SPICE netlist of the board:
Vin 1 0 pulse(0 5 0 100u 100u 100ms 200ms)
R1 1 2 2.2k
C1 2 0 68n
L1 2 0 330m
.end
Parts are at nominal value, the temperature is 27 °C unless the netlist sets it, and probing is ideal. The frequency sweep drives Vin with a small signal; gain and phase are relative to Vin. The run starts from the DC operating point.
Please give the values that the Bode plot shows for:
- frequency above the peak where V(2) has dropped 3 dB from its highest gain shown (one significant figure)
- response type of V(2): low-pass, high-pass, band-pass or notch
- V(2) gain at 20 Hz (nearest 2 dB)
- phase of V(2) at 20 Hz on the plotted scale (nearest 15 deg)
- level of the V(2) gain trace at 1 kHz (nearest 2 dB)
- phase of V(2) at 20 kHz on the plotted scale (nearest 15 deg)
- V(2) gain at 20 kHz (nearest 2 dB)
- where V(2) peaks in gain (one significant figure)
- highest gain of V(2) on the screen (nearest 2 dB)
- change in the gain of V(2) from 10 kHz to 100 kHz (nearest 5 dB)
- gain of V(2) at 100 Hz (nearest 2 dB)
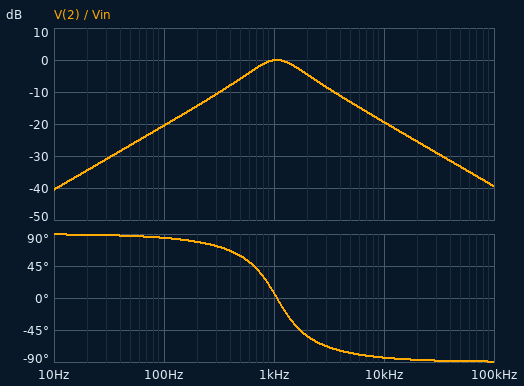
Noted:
2 kHz
band-pass
-34 dB
90 deg
0 dB
-90 deg
-26 dB
1 kHz
0 dB
-20 dB
-20 dB
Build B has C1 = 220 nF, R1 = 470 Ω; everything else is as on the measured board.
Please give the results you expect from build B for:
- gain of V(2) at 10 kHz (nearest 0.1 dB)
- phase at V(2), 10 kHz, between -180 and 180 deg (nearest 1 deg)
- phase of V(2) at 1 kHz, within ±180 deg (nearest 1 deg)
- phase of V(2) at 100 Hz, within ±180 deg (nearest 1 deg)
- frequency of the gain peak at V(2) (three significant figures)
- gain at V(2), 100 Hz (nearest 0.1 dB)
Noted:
-16.3 dB
-81 deg
-23 deg
66 deg
591 Hz
-7.7 dB
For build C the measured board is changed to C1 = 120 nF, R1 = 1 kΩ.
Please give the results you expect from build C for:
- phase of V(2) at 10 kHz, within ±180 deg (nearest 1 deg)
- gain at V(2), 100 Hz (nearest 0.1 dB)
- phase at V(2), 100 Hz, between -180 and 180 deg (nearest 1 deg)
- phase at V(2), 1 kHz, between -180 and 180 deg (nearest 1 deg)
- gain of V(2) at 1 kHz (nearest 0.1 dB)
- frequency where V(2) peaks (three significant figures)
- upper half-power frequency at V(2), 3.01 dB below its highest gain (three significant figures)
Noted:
-82 deg
-13.7 dB
78 deg
-15 deg
-0.3 dB
800 Hz
1.70 kHz
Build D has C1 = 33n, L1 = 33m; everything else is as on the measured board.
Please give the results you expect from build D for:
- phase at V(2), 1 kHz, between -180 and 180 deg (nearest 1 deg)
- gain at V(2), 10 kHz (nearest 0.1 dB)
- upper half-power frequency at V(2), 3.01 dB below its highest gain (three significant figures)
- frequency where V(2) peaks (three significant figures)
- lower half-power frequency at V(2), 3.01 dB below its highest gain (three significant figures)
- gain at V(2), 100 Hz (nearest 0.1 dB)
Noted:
84 deg
-11.2 dB
6.04 kHz
4.82 kHz
3.85 kHz
-40.5 dB
